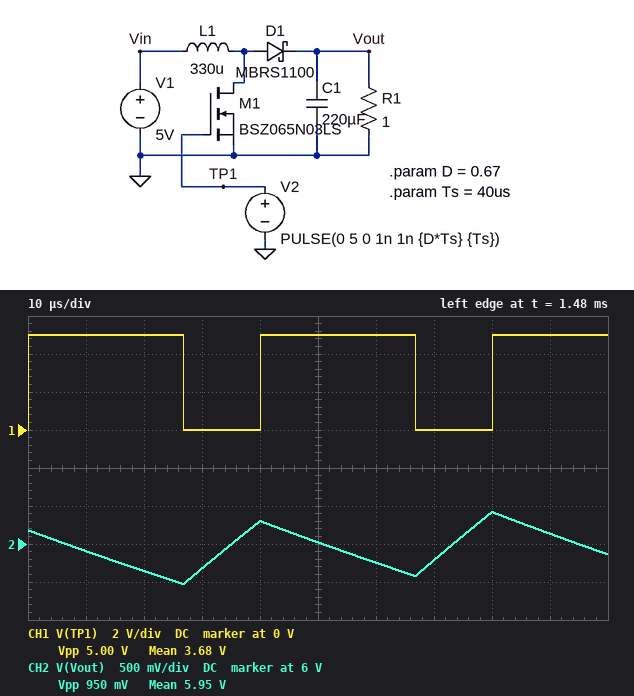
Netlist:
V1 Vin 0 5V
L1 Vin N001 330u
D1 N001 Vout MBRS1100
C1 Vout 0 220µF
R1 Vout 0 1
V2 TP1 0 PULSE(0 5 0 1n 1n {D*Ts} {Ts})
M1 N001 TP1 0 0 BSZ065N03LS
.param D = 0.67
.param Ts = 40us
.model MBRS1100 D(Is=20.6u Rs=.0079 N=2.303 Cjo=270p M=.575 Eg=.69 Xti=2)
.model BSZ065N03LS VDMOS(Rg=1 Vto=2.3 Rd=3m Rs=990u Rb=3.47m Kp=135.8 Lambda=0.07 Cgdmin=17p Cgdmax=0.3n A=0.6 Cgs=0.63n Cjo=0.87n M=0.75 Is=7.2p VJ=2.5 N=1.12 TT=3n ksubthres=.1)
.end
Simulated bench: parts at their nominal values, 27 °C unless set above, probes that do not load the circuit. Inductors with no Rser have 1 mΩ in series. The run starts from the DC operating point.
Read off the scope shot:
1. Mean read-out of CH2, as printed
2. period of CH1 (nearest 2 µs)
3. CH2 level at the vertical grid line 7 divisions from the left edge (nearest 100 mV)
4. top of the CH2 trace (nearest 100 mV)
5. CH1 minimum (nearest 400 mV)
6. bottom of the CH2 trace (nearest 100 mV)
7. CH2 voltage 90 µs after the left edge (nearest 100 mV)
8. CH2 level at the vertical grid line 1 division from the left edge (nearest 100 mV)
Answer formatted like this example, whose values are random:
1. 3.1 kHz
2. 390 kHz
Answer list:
1. 5.95 V
2. 40 µs
3. 5.8 V
4. 6.4 V
5. 0 V
6. 5.5 V
7. 6.1 V
8. 5.9 V
